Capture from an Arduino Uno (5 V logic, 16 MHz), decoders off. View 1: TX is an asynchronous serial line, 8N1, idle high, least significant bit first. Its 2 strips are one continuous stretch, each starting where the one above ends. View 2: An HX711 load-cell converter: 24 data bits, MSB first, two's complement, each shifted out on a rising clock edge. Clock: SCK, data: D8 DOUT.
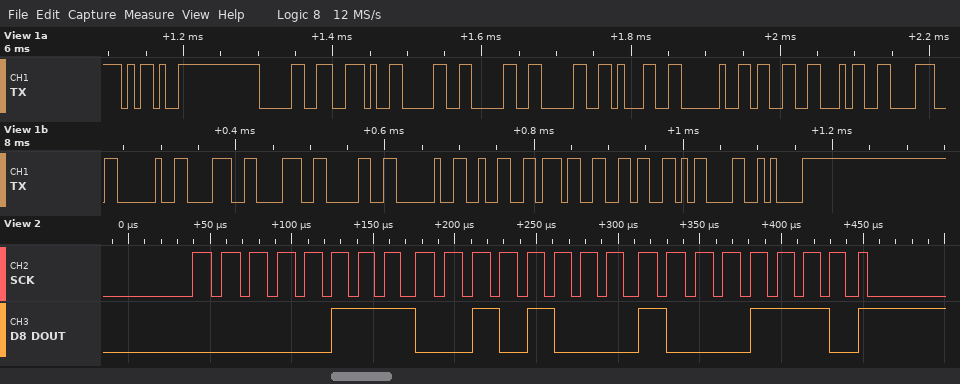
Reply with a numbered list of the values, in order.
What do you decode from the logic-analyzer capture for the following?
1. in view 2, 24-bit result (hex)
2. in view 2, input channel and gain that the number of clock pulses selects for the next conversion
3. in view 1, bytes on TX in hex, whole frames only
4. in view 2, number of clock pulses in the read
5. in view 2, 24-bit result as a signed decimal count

1. 0x07288E
2. channel A, gain 128
3. 2D 30 2E 30 30 30 31 20 33 34 38 20 38 38 30 20 32 37 36 0D 0A
4. 25
5. 469134
